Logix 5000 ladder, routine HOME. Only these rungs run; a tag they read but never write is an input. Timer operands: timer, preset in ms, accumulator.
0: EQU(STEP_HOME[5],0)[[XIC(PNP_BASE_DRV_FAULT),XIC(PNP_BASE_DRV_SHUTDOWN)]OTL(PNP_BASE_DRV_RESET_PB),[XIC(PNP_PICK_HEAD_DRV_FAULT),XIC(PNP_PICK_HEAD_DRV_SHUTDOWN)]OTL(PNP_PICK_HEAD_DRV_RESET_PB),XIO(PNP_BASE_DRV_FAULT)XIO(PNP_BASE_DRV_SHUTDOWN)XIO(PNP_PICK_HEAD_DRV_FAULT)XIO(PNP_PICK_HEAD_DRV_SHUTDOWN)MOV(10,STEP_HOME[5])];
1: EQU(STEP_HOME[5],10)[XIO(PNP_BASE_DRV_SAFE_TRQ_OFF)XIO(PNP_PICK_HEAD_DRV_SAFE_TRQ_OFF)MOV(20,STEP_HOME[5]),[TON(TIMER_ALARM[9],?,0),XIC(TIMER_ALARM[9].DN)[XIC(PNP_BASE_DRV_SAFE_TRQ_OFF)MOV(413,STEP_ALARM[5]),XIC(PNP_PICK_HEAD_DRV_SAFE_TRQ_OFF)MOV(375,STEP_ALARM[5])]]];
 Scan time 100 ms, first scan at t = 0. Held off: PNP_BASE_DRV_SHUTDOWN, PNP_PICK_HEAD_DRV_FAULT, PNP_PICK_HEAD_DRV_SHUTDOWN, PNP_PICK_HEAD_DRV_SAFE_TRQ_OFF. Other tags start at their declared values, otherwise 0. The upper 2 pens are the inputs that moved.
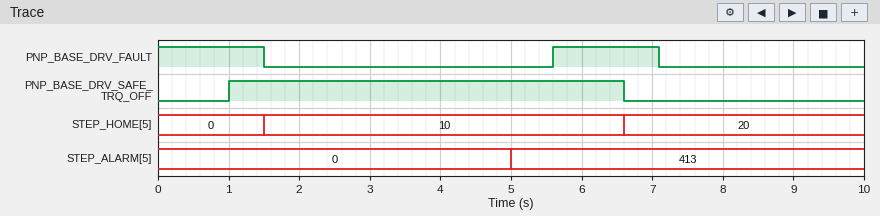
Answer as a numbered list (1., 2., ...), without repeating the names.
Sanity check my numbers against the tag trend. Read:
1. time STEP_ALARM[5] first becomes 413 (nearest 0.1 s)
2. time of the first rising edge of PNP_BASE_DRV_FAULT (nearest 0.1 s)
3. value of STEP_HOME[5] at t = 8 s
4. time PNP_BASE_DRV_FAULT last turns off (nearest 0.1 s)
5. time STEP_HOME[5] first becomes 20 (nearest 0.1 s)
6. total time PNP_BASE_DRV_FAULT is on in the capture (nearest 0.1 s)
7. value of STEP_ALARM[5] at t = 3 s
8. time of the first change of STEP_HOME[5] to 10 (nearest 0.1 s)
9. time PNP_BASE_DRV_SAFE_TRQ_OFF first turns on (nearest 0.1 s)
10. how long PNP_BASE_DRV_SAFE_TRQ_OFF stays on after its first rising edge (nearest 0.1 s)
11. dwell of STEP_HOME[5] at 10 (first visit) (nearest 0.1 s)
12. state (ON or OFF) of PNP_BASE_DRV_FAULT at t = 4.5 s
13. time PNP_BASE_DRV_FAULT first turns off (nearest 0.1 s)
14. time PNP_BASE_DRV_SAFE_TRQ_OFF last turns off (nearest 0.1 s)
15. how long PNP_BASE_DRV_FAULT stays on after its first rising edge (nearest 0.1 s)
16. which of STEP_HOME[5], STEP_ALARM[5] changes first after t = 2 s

1. 5.0 s
2. 5.6 s
3. 20
4. 7.1 s
5. 6.6 s
6. 3.0 s
7. 0
8. 1.5 s
9. 1.0 s
10. 5.6 s
11. 5.1 s
12. OFF
13. 1.5 s
14. 6.6 s
15. 1.5 s
16. STEP_ALARM[5]
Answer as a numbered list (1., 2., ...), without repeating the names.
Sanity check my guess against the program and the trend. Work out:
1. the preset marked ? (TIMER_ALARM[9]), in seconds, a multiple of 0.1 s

1. 3.5 s
